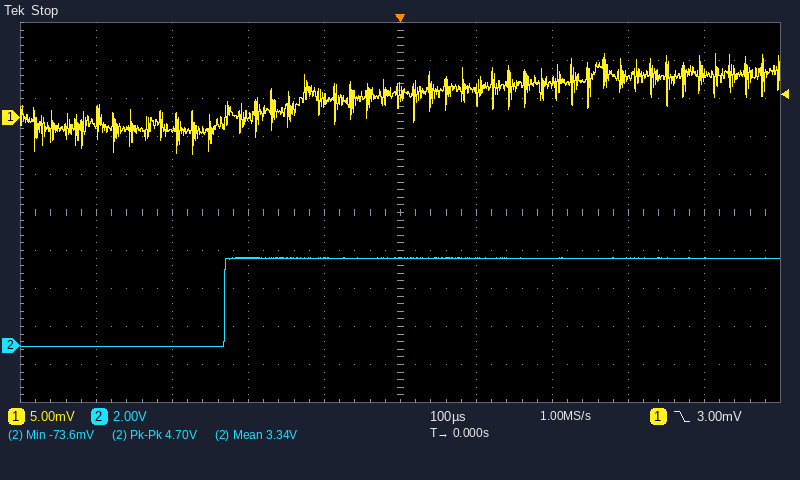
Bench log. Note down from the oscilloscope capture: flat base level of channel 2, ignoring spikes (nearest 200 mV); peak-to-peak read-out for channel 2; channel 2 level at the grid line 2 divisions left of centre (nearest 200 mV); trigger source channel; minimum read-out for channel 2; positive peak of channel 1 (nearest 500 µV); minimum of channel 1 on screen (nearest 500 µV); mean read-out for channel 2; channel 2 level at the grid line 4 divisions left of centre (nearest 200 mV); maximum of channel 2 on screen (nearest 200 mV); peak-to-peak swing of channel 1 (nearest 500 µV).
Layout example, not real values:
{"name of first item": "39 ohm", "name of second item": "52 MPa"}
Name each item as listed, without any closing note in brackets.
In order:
{"flat base level of channel 2, ignoring spikes": "0.0 V", "peak-to-peak read-out for channel 2": "4.70 V", "channel 2 level at the grid line 2 divisions left of centre": "4.6 V", "trigger source channel": "channel 1", "minimum read-out for channel 2": "-73.6 mV", "positive peak of channel 1": "8.5 mV", "minimum of channel 1 on screen": "-5.0 mV", "mean read-out for channel 2": "3.34 V", "channel 2 level at the grid line 4 divisions left of centre": "0.0 V", "maximum of channel 2 on screen": "4.6 V", "peak-to-peak swing of channel 1": "13.5 mV"}
